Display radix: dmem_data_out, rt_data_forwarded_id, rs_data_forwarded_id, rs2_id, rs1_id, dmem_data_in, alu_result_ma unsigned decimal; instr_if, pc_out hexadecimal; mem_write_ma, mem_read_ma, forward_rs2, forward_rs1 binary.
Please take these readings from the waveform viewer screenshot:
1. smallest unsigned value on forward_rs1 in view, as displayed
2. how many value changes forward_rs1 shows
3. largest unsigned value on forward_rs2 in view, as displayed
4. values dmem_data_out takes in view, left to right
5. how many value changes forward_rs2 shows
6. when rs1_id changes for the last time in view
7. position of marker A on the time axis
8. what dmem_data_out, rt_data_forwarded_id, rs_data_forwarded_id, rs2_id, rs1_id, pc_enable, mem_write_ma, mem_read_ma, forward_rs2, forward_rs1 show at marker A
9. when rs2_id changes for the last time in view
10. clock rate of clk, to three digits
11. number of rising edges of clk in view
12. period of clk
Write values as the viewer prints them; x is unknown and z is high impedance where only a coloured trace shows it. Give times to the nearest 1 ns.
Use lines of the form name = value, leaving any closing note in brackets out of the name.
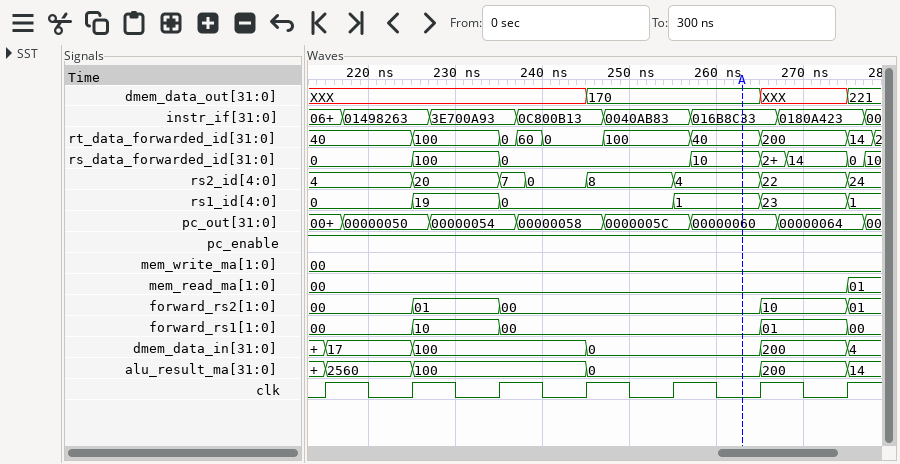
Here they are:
smallest unsigned value on forward_rs1 in view, as displayed = 00
how many value changes forward_rs1 shows = 4
largest unsigned value on forward_rs2 in view, as displayed = 10
values dmem_data_out takes in view, left to right = XXX, 170, XXX, 221
how many value changes forward_rs2 shows = 4
when rs1_id changes for the last time in view = 275 ns
position of marker A on the time axis = 263 ns
what dmem_data_out, rt_data_forwarded_id, rs_data_forwarded_id, rs2_id, rs1_id, pc_enable, mem_write_ma, mem_read_ma, forward_rs2, forward_rs1 show at marker A = dmem_data_out=170, rt_data_forwarded_id=40, rs_data_forwarded_id=10, rs2_id=4, rs1_id=1, pc_enable=1, mem_write_ma=00, mem_read_ma=00, forward_rs2=00, forward_rs1=00
when rs2_id changes for the last time in view = 275 ns
clock rate of clk, to three digits = 100 MHz
number of rising edges of clk in view = 7
period of clk = 10 ns
